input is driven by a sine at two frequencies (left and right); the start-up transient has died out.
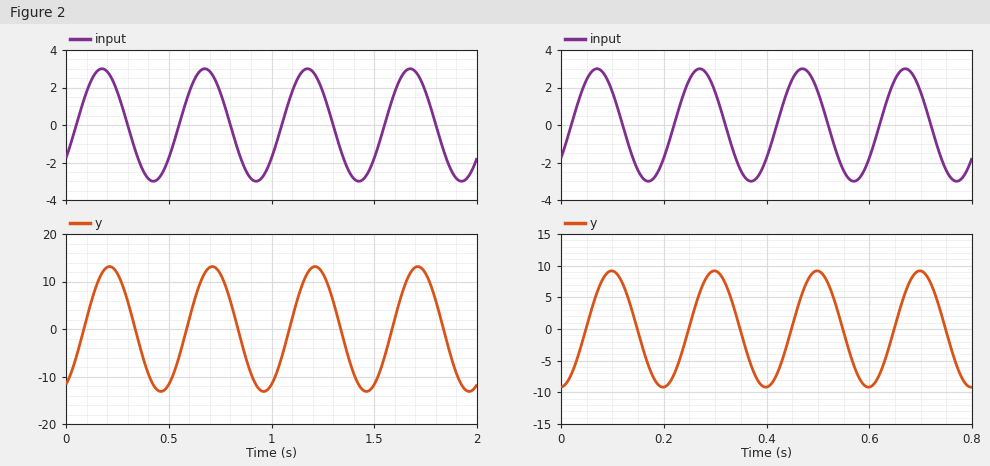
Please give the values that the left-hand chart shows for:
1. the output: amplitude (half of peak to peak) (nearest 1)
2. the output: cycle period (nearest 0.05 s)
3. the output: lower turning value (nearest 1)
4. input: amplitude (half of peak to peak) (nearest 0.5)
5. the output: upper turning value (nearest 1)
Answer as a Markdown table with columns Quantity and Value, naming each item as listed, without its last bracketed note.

| Quantity | Value |
|---|---|
| the output: amplitude (half of peak to peak) | 13 |
| the output: cycle period | 0.50 s |
| the output: lower turning value | -13 |
| input: amplitude (half of peak to peak) | 3.0 |
| the output: upper turning value | 13 |
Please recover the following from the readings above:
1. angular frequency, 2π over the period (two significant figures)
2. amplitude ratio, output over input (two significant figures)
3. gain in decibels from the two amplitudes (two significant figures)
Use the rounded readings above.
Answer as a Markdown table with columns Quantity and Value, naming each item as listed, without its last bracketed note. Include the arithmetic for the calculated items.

| Quantity | Value |
|---|---|
| angular frequency, 2π over the period | 2π / 0.5 = 13 rad/s |
| amplitude ratio, output over input | 13 / 3 = 4.3 |
| gain in decibels from the two amplitudes | 20 log10(13 / 3) = 13 dB |
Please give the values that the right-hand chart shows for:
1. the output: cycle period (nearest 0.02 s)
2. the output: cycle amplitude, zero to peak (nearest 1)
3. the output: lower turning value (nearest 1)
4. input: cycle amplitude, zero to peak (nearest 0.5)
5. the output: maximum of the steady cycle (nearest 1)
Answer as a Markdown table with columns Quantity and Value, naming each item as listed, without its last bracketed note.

| Quantity | Value |
|---|---|
| the output: cycle period | 0.20 s |
| the output: cycle amplitude, zero to peak | 9 |
| the output: lower turning value | -9 |
| input: cycle amplitude, zero to peak | 3.0 |
| the output: maximum of the steady cycle | 9 |
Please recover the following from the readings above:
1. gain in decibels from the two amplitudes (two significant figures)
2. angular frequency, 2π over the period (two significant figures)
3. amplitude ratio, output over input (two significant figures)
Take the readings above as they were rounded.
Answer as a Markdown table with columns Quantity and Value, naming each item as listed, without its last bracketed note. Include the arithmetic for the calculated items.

| Quantity | Value |
|---|---|
| gain in decibels from the two amplitudes | 20 log10(9 / 3) = 9.5 dB |
| angular frequency, 2π over the period | 2π / 0.2 = 31 rad/s |
| amplitude ratio, output over input | 9 / 3 = 3.0 |
